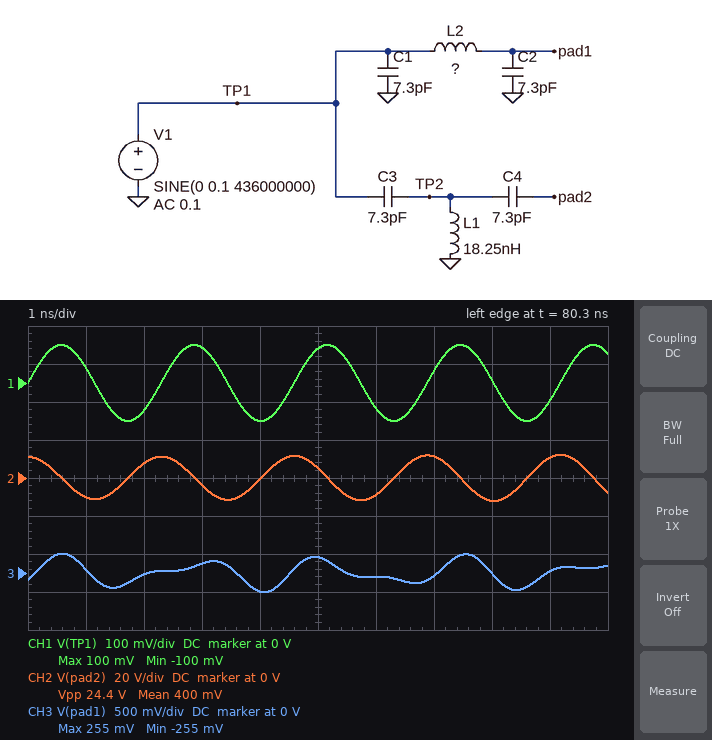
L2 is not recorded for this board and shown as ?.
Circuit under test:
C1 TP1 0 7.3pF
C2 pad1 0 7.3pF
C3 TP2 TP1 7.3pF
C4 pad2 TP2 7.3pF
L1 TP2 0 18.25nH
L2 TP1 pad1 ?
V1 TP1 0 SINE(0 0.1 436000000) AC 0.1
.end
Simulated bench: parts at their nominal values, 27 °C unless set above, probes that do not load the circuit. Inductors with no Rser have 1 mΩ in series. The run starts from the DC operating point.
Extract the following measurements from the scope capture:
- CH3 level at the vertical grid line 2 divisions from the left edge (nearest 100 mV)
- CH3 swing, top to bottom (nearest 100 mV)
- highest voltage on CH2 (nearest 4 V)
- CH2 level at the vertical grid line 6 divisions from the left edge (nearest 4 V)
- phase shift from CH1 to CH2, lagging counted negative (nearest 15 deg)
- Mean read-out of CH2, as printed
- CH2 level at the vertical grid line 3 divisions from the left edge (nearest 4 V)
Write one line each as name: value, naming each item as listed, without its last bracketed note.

CH3 level at the vertical grid line 2 divisions from the left edge: 0 V
CH3 swing, top to bottom: 500 mV
highest voltage on CH2: 12 V
CH2 level at the vertical grid line 6 divisions from the left edge: -8 V
phase shift from CH1 to CH2, lagging counted negative: 90 deg
Mean read-out of CH2, as printed: 400 mV
CH2 level at the vertical grid line 3 divisions from the left edge: -4 V
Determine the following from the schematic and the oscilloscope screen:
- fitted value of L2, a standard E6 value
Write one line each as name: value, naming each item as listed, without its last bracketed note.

fitted value of L2, a standard E6 value: 6.8 nH
